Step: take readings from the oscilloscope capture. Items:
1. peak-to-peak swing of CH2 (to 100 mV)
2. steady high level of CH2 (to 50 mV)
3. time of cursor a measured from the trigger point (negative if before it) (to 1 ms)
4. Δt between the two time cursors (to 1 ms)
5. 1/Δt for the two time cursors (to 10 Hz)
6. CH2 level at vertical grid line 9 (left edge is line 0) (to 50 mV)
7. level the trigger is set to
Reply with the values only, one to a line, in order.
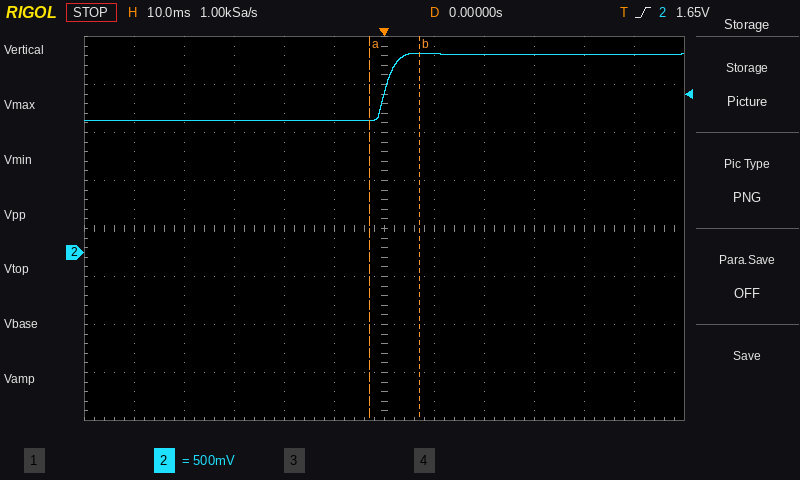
700 mV
2.05 V
-3 ms
10 ms
100 Hz
2.05 V
1.65 V
